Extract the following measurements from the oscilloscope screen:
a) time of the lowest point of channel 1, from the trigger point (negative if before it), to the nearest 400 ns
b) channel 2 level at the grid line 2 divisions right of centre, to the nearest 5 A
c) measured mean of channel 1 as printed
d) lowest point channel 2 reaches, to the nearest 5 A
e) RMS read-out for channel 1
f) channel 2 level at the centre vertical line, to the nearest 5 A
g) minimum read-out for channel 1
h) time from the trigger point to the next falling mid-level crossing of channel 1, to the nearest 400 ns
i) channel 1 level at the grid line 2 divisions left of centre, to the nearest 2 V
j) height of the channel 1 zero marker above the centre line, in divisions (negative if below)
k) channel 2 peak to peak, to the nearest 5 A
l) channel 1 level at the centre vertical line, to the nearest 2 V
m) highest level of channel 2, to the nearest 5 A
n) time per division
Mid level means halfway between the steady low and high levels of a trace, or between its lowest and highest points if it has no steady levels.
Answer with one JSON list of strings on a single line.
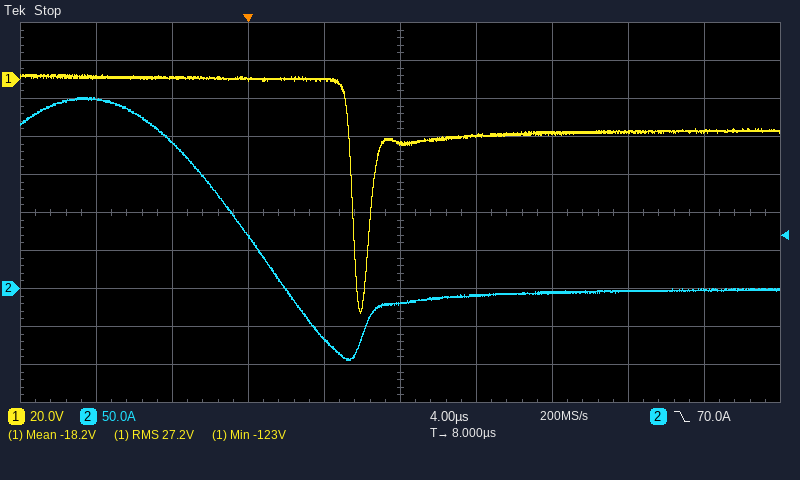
["+6.0 µs", "-5 A", "-18.2 V", "-95 A", "27.2 V", "-20 A", "-123 V", "5.6 µs", "0 V", "+3.5 div", "345 A", "-34 V", "250 A", "4 µs"]
